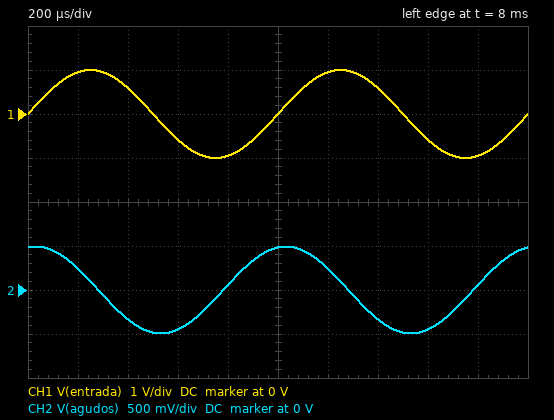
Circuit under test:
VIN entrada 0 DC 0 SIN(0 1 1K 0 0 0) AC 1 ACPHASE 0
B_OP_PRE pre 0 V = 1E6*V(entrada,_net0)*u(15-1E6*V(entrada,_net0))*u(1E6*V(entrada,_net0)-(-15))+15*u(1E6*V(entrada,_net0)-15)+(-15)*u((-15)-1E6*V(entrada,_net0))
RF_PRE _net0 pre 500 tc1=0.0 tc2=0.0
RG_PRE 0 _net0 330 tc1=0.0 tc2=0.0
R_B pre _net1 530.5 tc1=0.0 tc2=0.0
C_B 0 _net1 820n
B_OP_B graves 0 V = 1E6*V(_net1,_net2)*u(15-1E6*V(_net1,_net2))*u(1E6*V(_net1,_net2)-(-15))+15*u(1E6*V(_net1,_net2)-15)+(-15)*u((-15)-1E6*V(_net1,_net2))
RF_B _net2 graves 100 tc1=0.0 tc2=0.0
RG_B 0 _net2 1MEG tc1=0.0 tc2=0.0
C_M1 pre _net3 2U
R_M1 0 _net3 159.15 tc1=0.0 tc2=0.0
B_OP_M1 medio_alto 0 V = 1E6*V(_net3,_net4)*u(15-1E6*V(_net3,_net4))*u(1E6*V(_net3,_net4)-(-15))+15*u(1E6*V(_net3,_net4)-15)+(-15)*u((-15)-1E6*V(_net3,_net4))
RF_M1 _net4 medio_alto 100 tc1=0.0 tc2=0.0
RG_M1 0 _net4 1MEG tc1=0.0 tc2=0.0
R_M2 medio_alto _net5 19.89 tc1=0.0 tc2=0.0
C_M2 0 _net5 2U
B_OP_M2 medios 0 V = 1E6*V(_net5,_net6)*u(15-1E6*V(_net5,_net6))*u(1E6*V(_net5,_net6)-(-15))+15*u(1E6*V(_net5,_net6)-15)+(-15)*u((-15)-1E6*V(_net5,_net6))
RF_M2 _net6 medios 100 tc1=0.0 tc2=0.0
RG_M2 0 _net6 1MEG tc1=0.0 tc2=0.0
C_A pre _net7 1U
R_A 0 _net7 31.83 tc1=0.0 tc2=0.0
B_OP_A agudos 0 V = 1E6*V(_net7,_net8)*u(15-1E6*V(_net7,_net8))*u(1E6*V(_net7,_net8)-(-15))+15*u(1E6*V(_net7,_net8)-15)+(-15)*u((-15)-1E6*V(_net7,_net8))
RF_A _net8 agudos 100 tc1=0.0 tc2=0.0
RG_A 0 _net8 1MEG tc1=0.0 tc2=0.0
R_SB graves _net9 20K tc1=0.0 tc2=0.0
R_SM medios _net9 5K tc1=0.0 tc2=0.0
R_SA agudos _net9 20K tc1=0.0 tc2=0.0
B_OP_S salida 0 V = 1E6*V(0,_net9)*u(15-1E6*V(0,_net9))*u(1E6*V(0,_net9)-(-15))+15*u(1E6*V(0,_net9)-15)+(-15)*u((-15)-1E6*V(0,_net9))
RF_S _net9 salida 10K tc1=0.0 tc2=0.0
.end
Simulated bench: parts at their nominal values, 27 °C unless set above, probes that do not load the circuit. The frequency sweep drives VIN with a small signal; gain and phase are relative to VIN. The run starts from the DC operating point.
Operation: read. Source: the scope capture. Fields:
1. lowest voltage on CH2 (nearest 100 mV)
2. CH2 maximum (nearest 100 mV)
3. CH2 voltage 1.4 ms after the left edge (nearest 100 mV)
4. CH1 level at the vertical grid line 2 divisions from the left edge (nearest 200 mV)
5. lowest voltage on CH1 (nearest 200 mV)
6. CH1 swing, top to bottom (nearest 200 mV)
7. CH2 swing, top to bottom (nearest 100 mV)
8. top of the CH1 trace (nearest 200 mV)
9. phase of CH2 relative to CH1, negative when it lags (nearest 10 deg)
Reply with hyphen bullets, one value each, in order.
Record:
- -500 mV
- 500 mV
- -300 mV
- 600 mV
- -1.0 V
- 2.0 V
- 1.0 V
- 1.0 V
- 80 deg
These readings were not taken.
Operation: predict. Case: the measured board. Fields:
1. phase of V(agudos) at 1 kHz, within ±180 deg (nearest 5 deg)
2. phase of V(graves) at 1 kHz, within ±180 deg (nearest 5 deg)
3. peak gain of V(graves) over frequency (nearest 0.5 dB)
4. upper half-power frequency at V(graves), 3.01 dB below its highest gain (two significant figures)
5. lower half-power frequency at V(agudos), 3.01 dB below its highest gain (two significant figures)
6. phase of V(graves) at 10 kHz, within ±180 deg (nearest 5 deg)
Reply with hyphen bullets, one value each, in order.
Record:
- 80 deg
- -70 deg
- 8.0 dB
- 370 Hz
- 5.0 kHz
- -90 deg
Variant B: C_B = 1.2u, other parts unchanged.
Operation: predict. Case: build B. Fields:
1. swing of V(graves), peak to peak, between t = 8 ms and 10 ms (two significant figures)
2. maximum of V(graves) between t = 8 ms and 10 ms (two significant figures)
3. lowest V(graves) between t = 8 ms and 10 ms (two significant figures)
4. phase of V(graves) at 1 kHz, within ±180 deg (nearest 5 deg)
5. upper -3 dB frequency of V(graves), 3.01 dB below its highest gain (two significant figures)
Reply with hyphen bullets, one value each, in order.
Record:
- 1.2 V
- 610 mV
- -610 mV
- -75 deg
- 250 Hz
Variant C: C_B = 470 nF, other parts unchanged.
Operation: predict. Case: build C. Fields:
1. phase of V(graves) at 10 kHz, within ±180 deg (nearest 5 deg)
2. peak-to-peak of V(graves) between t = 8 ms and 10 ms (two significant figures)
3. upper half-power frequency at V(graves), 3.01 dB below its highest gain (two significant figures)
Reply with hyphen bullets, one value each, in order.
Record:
- -85 deg
- 2.7 V
- 640 Hz
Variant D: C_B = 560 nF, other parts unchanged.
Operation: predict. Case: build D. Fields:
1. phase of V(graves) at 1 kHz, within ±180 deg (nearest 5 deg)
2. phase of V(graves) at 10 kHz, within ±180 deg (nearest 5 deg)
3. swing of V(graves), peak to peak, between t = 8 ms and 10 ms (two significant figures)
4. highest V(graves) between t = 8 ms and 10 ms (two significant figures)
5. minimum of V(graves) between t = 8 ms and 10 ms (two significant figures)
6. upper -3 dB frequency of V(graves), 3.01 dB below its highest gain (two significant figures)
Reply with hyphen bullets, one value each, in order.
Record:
- -60 deg
- -85 deg
- 2.4 V
- 1.2 V
- -1.2 V
- 540 Hz
